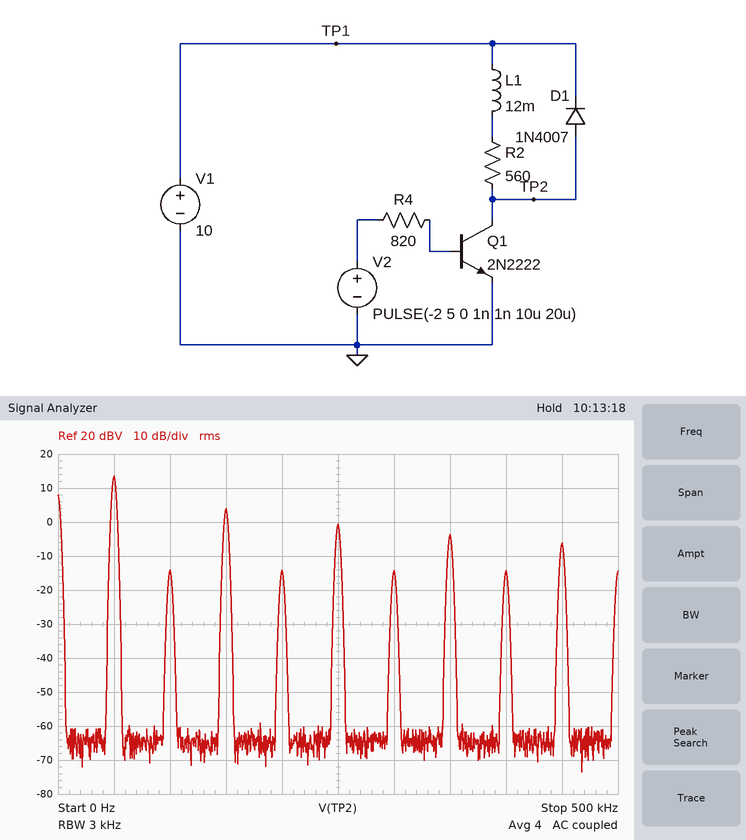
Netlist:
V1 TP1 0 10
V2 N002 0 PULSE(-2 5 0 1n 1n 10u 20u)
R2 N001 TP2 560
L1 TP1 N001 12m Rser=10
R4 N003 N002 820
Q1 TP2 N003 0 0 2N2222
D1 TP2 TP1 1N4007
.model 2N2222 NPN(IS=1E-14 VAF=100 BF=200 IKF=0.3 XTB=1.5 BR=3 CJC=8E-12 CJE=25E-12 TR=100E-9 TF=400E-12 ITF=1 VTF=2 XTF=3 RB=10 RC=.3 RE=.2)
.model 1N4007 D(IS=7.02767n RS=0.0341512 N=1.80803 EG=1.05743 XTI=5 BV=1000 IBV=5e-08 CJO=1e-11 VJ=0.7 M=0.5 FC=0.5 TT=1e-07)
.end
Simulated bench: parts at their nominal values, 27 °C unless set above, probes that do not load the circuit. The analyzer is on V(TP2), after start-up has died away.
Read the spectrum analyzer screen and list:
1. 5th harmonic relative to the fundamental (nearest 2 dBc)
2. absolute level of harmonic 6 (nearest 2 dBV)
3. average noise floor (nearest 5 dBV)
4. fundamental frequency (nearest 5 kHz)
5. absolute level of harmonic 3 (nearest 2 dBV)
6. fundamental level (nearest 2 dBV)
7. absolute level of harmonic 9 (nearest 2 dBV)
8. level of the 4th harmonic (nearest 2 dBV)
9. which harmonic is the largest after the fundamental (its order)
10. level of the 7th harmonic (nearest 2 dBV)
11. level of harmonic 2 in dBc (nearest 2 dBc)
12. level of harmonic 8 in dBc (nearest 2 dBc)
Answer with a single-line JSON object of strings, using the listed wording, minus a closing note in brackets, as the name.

{"5th harmonic relative to the fundamental": "-14 dBc", "absolute level of harmonic 6": "-14 dBV", "average noise floor": "-65 dBV", "fundamental frequency": "50 kHz", "absolute level of harmonic 3": "4 dBV", "fundamental level": "14 dBV", "absolute level of harmonic 9": "-6 dBV", "level of the 4th harmonic": "-14 dBV", "which harmonic is the largest after the fundamental": "3", "level of the 7th harmonic": "-4 dBV", "level of harmonic 2 in dBc": "-28 dBc", "level of harmonic 8 in dBc": "-28 dBc"}
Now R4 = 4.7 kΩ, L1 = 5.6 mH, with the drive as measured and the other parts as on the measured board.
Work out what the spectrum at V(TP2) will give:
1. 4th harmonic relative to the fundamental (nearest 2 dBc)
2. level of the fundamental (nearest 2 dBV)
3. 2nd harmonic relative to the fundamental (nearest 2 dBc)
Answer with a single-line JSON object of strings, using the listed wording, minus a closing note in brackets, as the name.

{"4th harmonic relative to the fundamental": "-30 dBc", "level of the fundamental": "14 dBV", "2nd harmonic relative to the fundamental": "-30 dBc"}
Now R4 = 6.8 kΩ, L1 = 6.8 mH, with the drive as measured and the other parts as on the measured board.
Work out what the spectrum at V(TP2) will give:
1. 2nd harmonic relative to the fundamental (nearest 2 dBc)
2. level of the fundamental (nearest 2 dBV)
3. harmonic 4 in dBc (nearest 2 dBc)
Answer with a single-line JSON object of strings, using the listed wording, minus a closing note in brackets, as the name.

{"2nd harmonic relative to the fundamental": "-32 dBc", "level of the fundamental": "14 dBV", "harmonic 4 in dBc": "-32 dBc"}
